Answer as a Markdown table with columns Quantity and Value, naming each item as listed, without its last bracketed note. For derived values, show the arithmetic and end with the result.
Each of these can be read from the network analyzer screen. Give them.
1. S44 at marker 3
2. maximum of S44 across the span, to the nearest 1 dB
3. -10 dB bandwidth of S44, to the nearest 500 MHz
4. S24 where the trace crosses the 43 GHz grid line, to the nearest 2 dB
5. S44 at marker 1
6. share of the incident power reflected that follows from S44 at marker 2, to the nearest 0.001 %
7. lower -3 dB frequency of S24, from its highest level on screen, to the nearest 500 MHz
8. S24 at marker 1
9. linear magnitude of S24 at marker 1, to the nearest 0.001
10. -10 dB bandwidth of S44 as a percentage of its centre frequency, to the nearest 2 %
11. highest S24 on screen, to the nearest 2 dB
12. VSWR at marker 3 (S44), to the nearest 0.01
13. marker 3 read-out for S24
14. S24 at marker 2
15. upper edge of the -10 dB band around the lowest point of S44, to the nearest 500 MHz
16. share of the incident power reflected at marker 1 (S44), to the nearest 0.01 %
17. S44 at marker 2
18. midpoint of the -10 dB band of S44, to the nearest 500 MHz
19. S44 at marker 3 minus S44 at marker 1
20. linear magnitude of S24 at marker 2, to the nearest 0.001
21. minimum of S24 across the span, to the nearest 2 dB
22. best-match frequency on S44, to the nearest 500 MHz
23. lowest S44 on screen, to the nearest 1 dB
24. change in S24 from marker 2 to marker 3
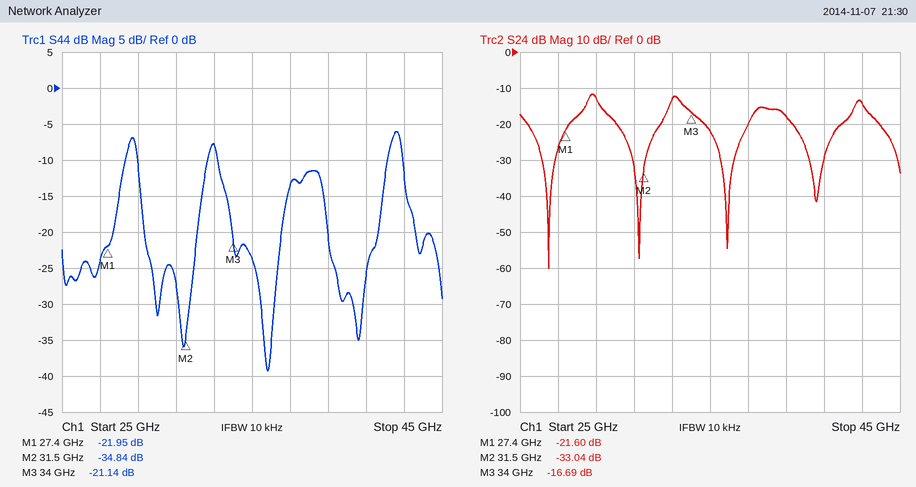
| Quantity | Value |
|---|---|
| S44 at marker 3 | -21.14 dB |
| maximum of S44 across the span, to the nearest 1 dB | -6 dB |
| -10 dB bandwidth of S44, to the nearest 500 MHz | 42.0 GHz − 33.0 GHz = 9.0 GHz |
| S24 where the trace crosses the 43 GHz grid line, to the nearest 2 dB | -14 dB |
| S44 at marker 1 | -21.95 dB |
| share of the incident power reflected that follows from S44 at marker 2, to the nearest 0.001 % | 10^(-34.84/10) ≈ 0.033 % |
| lower -3 dB frequency of S24, from its highest level on screen, to the nearest 500 MHz | 28.5 GHz |
| S24 at marker 1 | -21.60 dB |
| linear magnitude of S24 at marker 1, to the nearest 0.001 | 10^(-21.6/20) ≈ 0.083 |
| -10 dB bandwidth of S44 as a percentage of its centre frequency, to the nearest 2 % | 9 GHz / 37.5 GHz ≈ 24 % |
| highest S24 on screen, to the nearest 2 dB | -12 dB |
| VSWR at marker 3 (S44), to the nearest 0.01 | (1 + 0.0877)/(1 − 0.0877) ≈ 1.19 |
| marker 3 read-out for S24 | -16.69 dB |
| S24 at marker 2 | -33.04 dB |
| upper edge of the -10 dB band around the lowest point of S44, to the nearest 500 MHz | 42.0 GHz |
| share of the incident power reflected at marker 1 (S44), to the nearest 0.01 % | 10^(-21.95/10) ≈ 0.64 % |
| S44 at marker 2 | -34.84 dB |
| midpoint of the -10 dB band of S44, to the nearest 500 MHz | 37.5 GHz |
| S44 at marker 3 minus S44 at marker 1 | -21.14 − (-21.95) = 0.81 dB |
| linear magnitude of S24 at marker 2, to the nearest 0.001 | 10^(-33.04/20) ≈ 0.022 |
| minimum of S24 across the span, to the nearest 2 dB | -60 dB |
| best-match frequency on S44, to the nearest 500 MHz | 36.0 GHz |
| lowest S44 on screen, to the nearest 1 dB | -39 dB |
| change in S24 from marker 2 to marker 3 | -16.69 − (-33.04) = 16.35 dB |
